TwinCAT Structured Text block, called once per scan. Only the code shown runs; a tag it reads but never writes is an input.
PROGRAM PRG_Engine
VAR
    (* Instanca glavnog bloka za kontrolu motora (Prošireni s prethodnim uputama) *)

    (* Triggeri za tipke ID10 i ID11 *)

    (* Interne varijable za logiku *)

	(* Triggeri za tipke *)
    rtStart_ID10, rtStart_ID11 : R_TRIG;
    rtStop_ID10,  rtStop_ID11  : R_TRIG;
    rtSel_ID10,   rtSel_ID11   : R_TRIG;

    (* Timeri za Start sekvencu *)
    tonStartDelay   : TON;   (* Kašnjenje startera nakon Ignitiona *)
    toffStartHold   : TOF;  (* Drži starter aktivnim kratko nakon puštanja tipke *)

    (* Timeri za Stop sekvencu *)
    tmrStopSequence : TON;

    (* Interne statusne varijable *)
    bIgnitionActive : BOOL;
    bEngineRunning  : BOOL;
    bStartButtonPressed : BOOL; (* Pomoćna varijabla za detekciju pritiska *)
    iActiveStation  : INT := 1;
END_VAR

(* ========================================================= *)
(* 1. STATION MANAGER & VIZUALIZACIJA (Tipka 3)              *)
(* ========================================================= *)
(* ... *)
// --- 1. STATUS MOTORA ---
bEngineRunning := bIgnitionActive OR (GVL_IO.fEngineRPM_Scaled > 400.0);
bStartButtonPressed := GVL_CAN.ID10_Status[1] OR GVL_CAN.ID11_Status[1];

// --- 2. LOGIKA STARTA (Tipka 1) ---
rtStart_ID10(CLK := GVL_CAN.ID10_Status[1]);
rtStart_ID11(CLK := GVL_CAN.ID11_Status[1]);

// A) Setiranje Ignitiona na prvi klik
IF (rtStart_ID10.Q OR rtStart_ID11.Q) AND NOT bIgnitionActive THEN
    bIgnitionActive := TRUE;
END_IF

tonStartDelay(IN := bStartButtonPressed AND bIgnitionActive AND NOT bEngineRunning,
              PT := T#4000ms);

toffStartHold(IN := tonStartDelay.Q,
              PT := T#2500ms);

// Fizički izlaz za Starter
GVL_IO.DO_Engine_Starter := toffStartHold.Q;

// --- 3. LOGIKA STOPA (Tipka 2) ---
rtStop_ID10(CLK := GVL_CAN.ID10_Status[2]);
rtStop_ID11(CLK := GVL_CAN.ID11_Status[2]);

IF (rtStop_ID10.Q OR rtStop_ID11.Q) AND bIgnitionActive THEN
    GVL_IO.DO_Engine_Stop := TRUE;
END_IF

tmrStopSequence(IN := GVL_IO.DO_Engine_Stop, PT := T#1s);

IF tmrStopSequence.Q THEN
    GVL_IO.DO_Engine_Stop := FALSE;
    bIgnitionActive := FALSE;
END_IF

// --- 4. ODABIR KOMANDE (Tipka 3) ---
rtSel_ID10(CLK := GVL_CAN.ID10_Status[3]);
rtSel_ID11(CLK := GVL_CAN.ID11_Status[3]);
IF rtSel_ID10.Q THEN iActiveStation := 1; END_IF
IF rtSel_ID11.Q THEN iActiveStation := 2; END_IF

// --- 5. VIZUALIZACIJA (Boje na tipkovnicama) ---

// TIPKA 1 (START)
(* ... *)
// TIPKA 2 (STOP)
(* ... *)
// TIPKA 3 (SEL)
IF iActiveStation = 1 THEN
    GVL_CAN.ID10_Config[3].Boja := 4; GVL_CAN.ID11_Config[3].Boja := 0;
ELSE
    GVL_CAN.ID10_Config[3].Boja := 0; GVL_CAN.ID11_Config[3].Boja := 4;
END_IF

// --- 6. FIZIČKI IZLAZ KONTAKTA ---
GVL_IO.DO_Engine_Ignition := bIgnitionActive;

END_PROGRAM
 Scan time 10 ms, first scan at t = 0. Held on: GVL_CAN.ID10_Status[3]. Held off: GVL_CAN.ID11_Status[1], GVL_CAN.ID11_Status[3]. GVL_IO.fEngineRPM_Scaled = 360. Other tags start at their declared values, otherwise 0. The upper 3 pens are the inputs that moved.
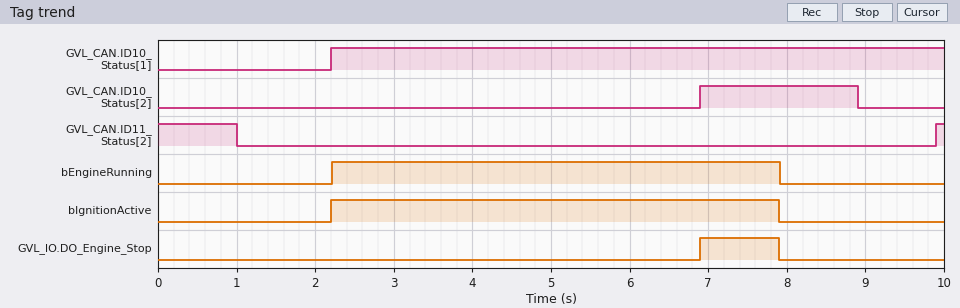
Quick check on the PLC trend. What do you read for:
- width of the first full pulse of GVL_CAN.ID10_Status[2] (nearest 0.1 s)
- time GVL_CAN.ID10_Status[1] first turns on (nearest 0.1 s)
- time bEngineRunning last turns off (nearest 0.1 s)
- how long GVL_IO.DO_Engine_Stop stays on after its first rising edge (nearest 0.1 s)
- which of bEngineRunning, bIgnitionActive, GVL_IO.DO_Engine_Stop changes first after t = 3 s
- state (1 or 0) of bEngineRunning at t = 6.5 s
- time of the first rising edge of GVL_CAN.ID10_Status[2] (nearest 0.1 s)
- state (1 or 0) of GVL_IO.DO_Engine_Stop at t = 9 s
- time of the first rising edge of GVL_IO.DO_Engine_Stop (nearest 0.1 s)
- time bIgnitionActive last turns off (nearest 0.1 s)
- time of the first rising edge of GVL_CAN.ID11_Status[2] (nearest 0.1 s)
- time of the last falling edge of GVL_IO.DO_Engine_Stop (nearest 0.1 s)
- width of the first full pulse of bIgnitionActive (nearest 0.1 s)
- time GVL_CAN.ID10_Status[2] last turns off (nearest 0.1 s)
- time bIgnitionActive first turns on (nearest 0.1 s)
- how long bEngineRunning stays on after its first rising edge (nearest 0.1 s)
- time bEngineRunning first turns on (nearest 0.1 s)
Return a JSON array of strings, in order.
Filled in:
["2.0 s", "2.2 s", "7.9 s", "1.0 s", "GVL_IO.DO_Engine_Stop", "1", "6.9 s", "0", "6.9 s", "7.9 s", "9.9 s", "7.9 s", "5.7 s", "8.9 s", "2.2 s", "5.7 s", "2.2 s"]
